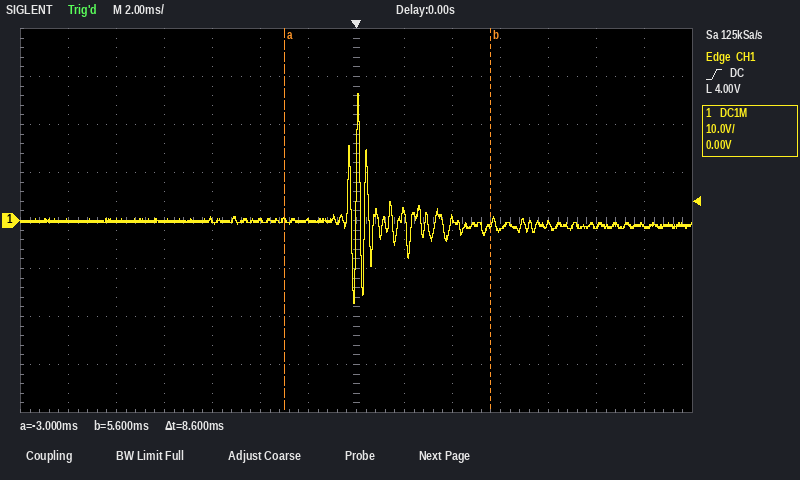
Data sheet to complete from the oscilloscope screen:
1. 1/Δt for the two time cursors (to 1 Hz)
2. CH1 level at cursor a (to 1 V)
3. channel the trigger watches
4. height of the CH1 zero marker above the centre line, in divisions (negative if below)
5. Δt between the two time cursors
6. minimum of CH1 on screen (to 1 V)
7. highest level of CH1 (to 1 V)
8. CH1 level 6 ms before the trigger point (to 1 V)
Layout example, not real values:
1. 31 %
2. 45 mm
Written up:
1. 116 Hz
2. 0 V
3. CH1
4. 0.0 div
5. 8.6 ms
6. -17 V
7. 26 V
8. 0 V
